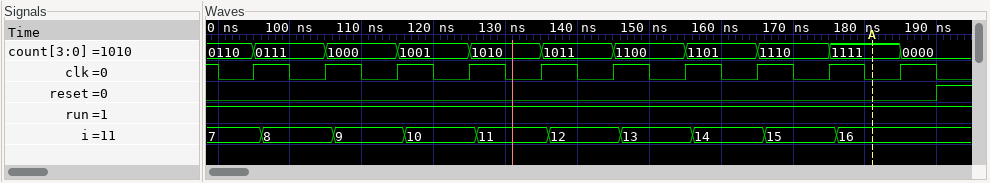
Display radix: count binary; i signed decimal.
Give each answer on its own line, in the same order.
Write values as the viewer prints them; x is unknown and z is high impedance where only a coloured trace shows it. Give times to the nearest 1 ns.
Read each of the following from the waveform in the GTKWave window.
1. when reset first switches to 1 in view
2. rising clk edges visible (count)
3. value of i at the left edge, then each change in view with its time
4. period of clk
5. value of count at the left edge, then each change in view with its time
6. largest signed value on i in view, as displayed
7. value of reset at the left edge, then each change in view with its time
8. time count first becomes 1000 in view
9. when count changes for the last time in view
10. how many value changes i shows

190 ns
10
7, 8 at 96 ns, 9 at 106 ns, 10 at 116 ns, 11 at 126 ns, 12 at 136 ns, 13 at 146 ns, 14 at 156 ns, 15 at 166 ns, 16 at 176 ns
10 ns
0110, 0111 at 95 ns, 1000 at 105 ns, 1001 at 115 ns, 1010 at 125 ns, 1011 at 135 ns, 1100 at 145 ns, 1101 at 155 ns, 1110 at 165 ns, 1111 at 175 ns, 0000 at 185 ns
16
0, 1 at 190 ns
105 ns
185 ns
9
